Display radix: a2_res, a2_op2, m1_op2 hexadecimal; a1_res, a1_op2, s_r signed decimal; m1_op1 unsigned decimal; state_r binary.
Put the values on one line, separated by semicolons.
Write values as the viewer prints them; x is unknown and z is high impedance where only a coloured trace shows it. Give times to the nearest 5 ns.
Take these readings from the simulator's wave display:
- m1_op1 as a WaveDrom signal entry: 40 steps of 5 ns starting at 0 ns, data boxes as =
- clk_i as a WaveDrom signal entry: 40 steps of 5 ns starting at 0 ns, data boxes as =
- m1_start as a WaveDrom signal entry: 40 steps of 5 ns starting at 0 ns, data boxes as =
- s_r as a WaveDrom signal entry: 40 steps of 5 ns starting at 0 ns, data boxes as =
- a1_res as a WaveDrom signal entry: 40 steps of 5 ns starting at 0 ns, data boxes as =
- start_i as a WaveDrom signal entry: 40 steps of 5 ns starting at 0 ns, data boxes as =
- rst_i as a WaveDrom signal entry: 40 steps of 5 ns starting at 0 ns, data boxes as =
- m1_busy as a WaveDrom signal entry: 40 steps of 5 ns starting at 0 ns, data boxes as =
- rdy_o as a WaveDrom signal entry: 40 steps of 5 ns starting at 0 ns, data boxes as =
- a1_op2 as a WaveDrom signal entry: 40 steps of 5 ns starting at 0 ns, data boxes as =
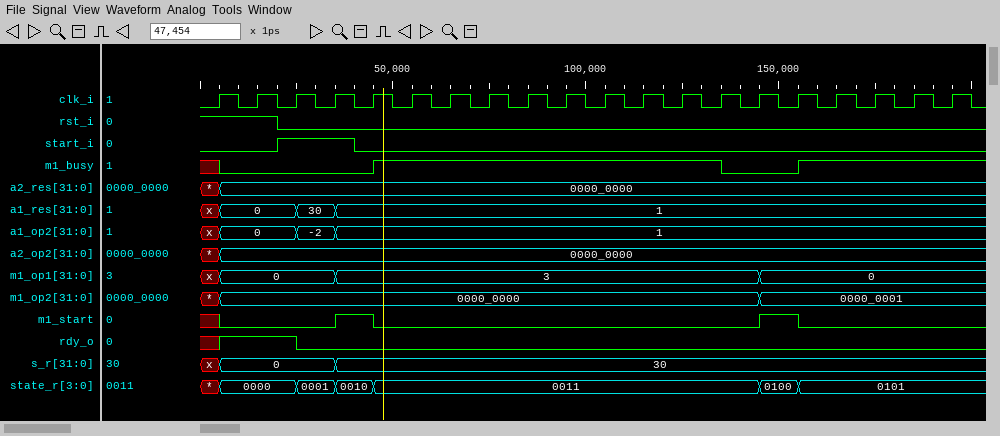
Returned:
{name: 'm1_op1', wave: 'x=.....=.....................=..........', data: '0 3 0'}; {name: 'clk_i', wave: '0101010101010101010101010101010101010101'}; {name: 'm1_start', wave: 'x0.....1.0...................1.0........'}; {name: 's_r', wave: 'x=.....=................................', data: '0 30'}; {name: 'a1_res', wave: 'x=...=.=................................', data: '0 30 1'}; {name: 'start_i', wave: '0...1...0...............................'}; {name: 'rst_i', wave: '1...0...................................'}; {name: 'm1_busy', wave: 'x0.......1.................0...1........'}; {name: 'rdy_o', wave: 'x1...0..................................'}; {name: 'a1_op2', wave: 'x=...=.=................................', data: '0 -2 1'}
